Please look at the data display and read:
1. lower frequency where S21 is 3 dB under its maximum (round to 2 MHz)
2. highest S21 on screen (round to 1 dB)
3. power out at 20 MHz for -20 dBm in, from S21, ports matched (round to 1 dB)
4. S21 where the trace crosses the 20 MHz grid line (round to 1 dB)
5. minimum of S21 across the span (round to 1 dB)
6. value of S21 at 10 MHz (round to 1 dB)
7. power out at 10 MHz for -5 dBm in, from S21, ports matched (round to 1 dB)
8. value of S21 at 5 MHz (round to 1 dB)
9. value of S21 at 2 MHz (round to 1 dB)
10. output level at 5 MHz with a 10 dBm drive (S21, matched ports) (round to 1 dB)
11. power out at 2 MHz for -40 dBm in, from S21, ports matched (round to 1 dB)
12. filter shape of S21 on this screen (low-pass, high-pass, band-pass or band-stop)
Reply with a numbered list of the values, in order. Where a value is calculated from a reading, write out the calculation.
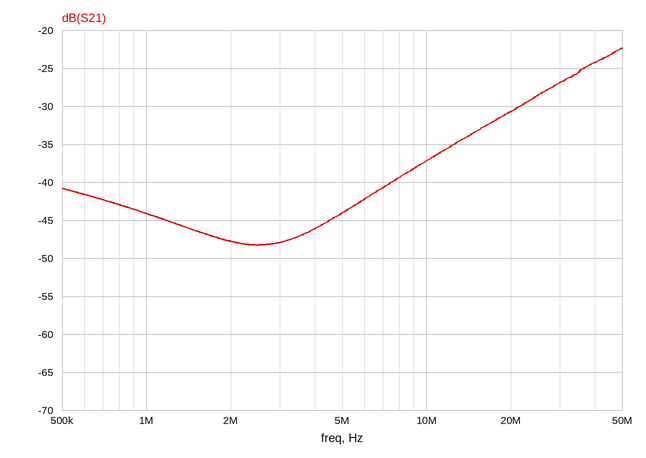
1. 36 MHz
2. -22 dB
3. -20 dBm + (-31 dB) = -51 dBm
4. -31 dB
5. -48 dB
6. -37 dB
7. -5 dBm + (-37 dB) = -42 dBm
8. -44 dB
9. -48 dB
10. 10 dBm + (-44 dB) = -34 dBm
11. -40 dBm + (-48 dB) = -88 dBm
12. high-pass
